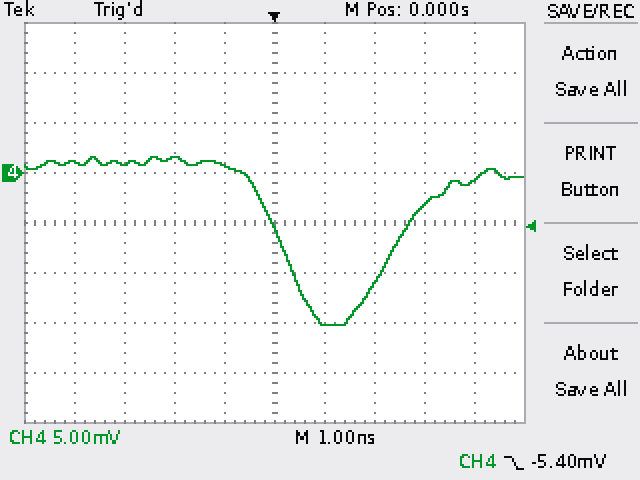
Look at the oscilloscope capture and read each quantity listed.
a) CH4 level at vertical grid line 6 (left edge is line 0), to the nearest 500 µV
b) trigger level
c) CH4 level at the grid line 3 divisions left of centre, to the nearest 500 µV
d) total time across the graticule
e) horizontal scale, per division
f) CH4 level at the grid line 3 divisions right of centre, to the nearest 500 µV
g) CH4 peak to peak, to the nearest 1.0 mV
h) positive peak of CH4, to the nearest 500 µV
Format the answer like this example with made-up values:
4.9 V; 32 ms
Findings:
-15.0 mV; -5.40 mV; 1.0 mV; 10 ns; 1 ns; -3.0 mV; 17.0 mV; 1.5 mV
